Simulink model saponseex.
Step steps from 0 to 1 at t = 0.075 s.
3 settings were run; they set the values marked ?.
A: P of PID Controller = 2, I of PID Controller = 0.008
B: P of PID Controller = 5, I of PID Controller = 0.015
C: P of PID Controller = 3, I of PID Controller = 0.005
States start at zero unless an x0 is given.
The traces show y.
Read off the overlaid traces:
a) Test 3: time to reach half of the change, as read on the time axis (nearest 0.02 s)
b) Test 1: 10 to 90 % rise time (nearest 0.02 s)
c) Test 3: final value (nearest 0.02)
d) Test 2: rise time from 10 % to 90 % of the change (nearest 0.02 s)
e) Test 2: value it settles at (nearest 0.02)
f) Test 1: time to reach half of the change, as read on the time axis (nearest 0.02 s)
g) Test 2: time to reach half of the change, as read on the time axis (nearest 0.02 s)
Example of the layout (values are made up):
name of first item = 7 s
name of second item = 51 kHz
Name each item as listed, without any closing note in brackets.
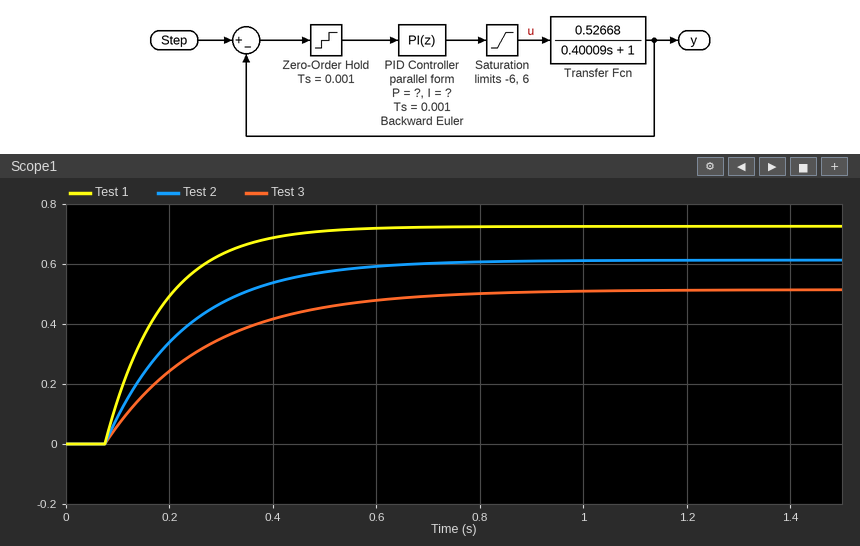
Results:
Test 3: time to reach half of the change, as read on the time axis = 0.22 s
Test 1: 10 to 90 % rise time = 0.24 s
Test 3: final value = 0.52
Test 2: rise time from 10 % to 90 % of the change = 0.34 s
Test 2: value it settles at = 0.62
Test 1: time to reach half of the change, as read on the time axis = 0.16 s
Test 2: time to reach half of the change, as read on the time axis = 0.18 s
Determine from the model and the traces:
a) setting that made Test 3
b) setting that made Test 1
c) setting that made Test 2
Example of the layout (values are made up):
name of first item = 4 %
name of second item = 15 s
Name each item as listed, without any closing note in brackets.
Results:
setting that made Test 3 = A
setting that made Test 1 = B
setting that made Test 2 = C
